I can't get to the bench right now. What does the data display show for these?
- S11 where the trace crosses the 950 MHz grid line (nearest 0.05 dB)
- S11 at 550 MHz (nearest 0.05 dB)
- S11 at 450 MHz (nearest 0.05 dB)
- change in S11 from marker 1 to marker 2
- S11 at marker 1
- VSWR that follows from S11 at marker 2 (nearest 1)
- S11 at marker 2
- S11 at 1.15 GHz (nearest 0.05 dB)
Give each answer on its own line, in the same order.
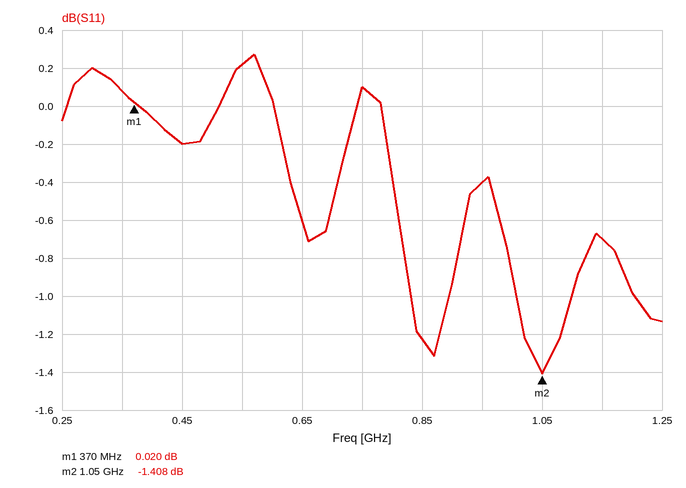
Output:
-0.40 dB
0.20 dB
-0.20 dB
-1.428 dB
0.020 dB
12
-1.408 dB
-0.70 dB
